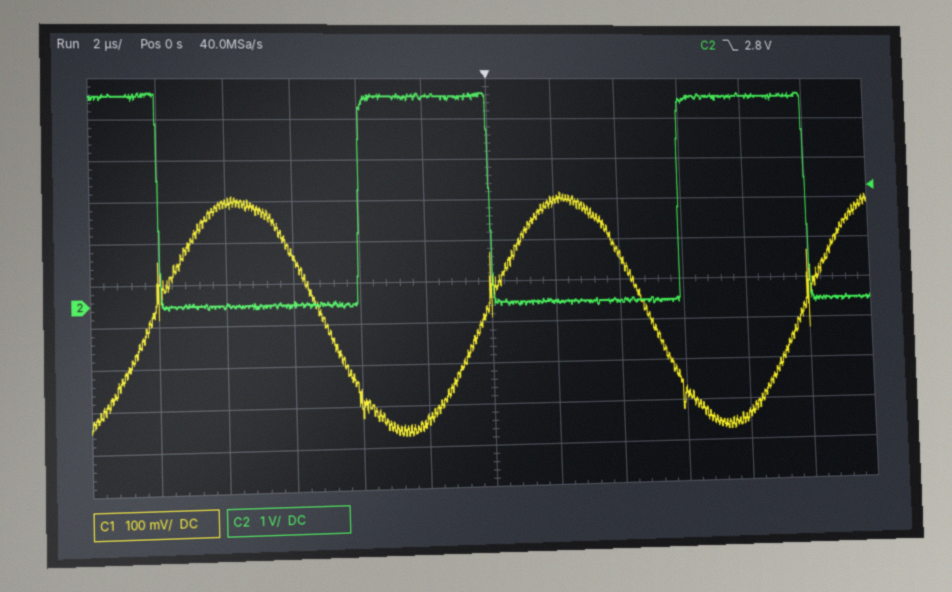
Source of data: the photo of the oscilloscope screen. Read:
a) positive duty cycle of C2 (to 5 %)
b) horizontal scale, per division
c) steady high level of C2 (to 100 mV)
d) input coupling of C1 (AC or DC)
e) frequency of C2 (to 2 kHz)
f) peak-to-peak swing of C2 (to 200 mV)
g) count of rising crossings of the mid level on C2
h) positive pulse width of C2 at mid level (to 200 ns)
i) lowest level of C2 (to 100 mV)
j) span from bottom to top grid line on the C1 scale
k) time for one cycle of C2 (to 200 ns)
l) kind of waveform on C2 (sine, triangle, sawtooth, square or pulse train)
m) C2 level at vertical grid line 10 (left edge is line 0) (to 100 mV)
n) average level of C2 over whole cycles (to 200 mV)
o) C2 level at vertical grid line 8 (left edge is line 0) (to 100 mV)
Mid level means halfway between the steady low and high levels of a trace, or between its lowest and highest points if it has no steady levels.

40 %
2 µs
5.1 V
DC
100 kHz
5.2 V
2
4.0 µs
-100 mV
1 V
10.0 µs
pulse train
5.1 V
2.0 V
0.0 V
